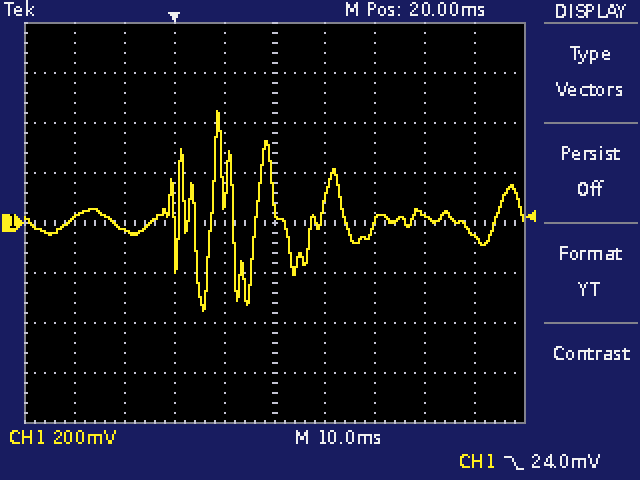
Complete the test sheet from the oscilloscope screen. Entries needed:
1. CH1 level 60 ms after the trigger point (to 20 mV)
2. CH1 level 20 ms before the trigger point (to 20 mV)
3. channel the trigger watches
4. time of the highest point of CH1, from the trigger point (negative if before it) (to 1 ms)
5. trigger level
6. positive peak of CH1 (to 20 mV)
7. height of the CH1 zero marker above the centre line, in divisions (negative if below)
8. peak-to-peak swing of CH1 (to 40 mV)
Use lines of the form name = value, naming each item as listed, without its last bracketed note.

CH1 level 60 ms after the trigger point = -60 mV
CH1 level 20 ms before the trigger point = 20 mV
channel the trigger watches = CH1
time of the highest point of CH1, from the trigger point (negative if before it) = +9 ms
trigger level = 24.0 mV
positive peak of CH1 = 440 mV
height of the CH1 zero marker above the centre line, in divisions = 0.0 div
peak-to-peak swing of CH1 = 800 mV
